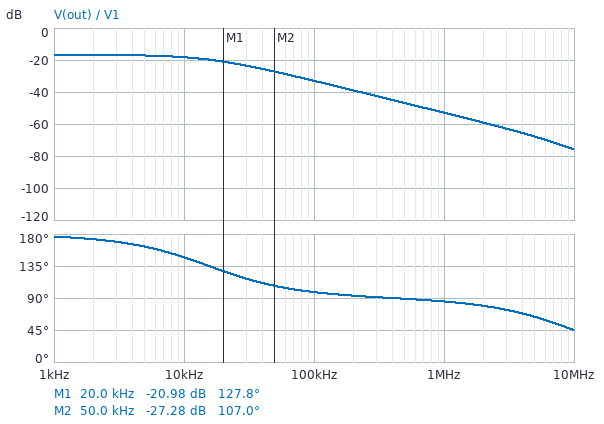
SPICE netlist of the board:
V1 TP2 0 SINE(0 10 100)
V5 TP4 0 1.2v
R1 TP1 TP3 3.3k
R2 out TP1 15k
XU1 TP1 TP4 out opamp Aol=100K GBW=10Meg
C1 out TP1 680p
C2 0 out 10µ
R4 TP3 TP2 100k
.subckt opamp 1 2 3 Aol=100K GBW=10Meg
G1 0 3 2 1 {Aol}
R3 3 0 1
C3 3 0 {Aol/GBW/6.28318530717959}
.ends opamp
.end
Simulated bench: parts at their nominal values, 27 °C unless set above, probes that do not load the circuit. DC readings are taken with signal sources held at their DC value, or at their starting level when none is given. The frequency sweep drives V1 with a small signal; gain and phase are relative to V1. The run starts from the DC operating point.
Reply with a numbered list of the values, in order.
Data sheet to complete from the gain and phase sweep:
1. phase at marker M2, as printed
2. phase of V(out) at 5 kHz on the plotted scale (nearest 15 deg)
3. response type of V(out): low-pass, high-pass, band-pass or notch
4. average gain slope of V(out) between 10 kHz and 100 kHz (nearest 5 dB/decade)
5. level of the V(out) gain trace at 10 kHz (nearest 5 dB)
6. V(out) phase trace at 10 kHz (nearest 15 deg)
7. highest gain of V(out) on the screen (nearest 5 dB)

1. 107.0 deg
2. 165 deg
3. low-pass
4. -15 dB/decade
5. -20 dB
6. 150 deg
7. -15 dB
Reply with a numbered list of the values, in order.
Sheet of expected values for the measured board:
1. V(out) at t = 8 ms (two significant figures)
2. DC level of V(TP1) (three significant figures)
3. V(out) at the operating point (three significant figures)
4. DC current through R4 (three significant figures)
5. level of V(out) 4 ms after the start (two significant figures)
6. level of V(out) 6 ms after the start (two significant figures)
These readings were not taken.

1. 2.8 V
2. 1.20 V
3. 1.37 V
4. 11.6 µA
5. 510 mV
6. 2.2 V
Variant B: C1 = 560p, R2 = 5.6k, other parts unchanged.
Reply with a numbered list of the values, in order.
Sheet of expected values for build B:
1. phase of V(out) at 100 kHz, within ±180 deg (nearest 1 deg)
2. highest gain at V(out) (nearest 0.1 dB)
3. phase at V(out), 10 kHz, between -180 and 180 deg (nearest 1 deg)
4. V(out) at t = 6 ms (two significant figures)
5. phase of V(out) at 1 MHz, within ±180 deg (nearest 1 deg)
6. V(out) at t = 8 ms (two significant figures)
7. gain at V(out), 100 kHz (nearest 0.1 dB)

1. 116 deg
2. -25.3 dB
3. 169 deg
4. 1.6 V
5. 87 deg
6. 1.8 V
7. -32.2 dB
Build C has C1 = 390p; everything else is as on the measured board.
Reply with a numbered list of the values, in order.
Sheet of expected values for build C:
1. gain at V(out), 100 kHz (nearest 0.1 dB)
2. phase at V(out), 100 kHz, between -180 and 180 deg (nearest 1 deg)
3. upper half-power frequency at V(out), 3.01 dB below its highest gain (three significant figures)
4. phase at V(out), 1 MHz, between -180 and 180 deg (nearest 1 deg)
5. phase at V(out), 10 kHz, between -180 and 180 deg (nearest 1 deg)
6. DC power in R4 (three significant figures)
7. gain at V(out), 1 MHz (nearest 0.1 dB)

1. -28.4 dB
2. 105 deg
3. 27.2 kHz
4. 86 deg
5. 160 deg
6. 13.5 µW
7. -48.1 dB
